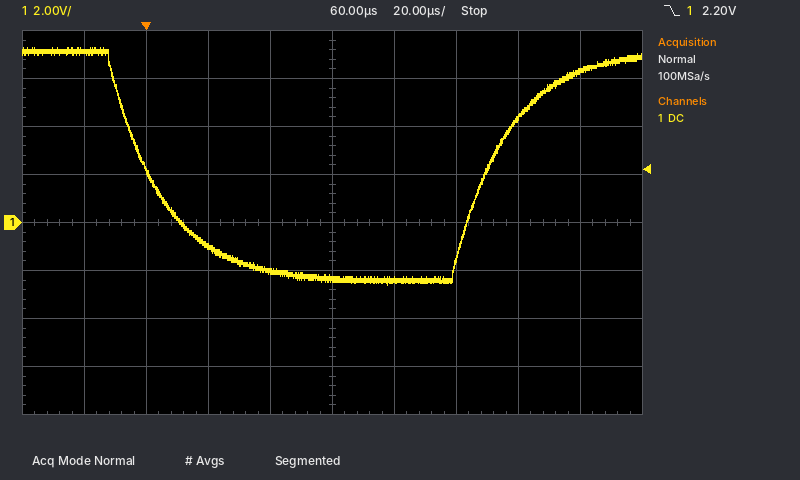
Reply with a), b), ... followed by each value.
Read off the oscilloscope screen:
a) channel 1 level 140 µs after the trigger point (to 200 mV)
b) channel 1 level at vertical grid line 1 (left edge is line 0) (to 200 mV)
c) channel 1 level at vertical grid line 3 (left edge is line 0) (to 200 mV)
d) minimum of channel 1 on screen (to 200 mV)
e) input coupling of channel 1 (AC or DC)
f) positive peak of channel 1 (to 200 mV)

a) 6.2 V
b) 7.0 V
c) -1.0 V
d) -2.6 V
e) DC
f) 7.2 V
